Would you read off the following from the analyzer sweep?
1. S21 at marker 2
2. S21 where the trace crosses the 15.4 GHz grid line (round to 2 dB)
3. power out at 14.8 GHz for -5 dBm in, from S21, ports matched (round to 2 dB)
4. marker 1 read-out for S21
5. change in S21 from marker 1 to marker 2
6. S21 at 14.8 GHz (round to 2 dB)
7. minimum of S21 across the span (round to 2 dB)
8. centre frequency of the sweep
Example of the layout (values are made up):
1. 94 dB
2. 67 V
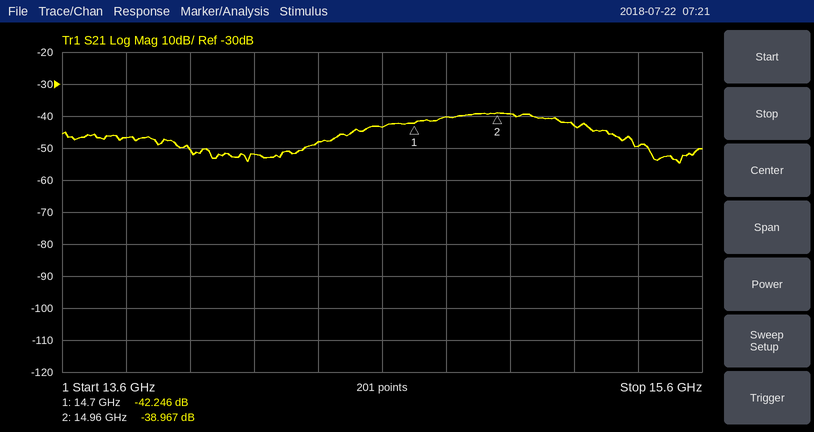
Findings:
1. -38.967 dB
2. -50 dB
3. -46 dBm
4. -42.246 dB
5. 3.279 dB
6. -40 dB
7. -54 dB
8. 14.6 GHz
